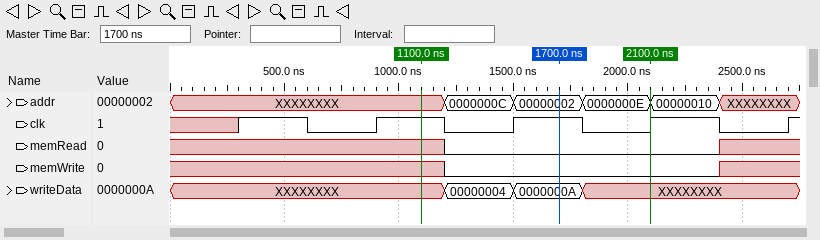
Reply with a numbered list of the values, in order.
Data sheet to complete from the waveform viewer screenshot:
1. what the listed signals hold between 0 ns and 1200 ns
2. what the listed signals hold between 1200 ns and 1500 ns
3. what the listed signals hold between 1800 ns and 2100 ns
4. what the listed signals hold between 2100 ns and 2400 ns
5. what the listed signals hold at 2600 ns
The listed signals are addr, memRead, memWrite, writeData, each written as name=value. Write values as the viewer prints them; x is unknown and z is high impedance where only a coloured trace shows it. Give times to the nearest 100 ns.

1. addr=XXXXXXXX, memRead=x, memWrite=x, writeData=XXXXXXXX
2. addr=0000000C, memRead=0, memWrite=0, writeData=00000004
3. addr=0000000E, memRead=0, memWrite=0, writeData=XXXXXXXX
4. addr=00000010, memRead=0, memWrite=0, writeData=XXXXXXXX
5. addr=XXXXXXXX, memRead=x, memWrite=x, writeData=XXXXXXXX
